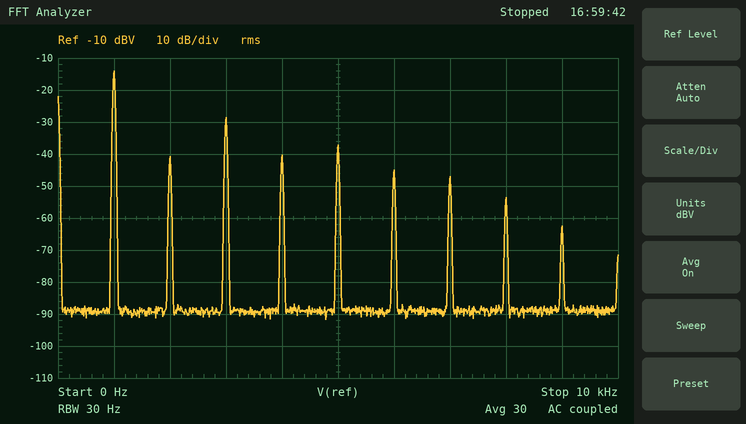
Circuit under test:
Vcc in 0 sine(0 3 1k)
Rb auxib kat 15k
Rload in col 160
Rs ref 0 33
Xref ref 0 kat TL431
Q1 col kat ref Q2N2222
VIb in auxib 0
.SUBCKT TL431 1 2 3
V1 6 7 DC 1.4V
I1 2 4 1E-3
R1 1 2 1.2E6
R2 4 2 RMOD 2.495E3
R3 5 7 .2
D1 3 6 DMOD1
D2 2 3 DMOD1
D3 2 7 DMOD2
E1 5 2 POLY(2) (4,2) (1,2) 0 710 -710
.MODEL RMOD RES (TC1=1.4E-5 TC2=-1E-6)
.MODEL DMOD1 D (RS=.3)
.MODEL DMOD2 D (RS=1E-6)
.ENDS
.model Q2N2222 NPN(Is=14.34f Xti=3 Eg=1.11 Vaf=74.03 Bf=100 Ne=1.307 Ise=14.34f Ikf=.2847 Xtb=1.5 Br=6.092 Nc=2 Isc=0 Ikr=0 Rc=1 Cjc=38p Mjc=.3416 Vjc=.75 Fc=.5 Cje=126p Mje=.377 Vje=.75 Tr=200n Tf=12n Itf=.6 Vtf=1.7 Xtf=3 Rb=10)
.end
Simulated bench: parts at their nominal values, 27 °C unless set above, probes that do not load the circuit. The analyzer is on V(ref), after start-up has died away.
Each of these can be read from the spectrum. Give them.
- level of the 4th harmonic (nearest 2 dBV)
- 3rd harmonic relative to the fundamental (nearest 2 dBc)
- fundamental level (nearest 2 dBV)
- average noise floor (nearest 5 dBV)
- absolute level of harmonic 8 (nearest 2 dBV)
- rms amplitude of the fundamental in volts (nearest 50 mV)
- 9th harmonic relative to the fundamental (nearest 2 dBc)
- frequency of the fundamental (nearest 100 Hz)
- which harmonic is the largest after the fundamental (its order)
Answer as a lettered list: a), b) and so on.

a) -40 dBV
b) -14 dBc
c) -14 dBV
d) -90 dBV
e) -54 dBV
f) 200 mV
g) -48 dBc
h) 1.0 kHz
i) 3
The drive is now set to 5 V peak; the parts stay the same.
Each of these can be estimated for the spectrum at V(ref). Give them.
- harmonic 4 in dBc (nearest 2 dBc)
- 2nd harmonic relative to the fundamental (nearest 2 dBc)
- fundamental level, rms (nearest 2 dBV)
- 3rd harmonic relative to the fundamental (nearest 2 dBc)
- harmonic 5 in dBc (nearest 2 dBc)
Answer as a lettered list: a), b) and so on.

a) -36 dBc
b) -46 dBc
c) -8 dBV
d) -20 dBc
e) -26 dBc
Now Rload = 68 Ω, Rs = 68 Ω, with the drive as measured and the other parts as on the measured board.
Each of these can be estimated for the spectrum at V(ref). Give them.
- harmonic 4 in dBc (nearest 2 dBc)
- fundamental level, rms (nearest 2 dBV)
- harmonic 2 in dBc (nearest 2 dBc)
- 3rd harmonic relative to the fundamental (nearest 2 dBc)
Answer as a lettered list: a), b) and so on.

a) -28 dBc
b) -4 dBV
c) -12 dBc
d) -12 dBc
